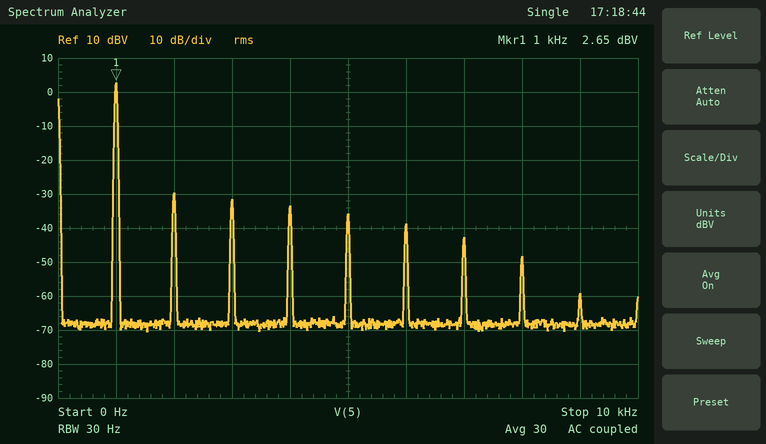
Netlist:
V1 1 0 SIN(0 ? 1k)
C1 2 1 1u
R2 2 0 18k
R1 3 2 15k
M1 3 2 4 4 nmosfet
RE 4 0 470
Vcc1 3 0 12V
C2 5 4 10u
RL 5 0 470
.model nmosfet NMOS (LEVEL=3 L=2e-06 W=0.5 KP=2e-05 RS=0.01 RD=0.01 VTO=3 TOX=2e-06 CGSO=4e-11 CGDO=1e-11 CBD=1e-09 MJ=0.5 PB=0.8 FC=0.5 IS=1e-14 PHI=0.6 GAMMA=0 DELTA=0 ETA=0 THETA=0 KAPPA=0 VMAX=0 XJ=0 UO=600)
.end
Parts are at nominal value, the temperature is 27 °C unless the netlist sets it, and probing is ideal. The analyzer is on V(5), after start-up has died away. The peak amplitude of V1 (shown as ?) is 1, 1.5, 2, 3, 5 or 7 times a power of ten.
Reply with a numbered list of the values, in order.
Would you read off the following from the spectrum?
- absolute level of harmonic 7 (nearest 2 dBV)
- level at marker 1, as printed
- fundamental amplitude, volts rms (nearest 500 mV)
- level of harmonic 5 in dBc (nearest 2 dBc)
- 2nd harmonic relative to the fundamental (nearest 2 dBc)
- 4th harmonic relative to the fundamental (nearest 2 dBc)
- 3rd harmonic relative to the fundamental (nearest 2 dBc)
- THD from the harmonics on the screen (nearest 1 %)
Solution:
1. -42 dBV
2. 2.65 dBV
3. 1.5 V
4. -38 dBc
5. -32 dBc
6. -36 dBc
7. -34 dBc
8. 4 %
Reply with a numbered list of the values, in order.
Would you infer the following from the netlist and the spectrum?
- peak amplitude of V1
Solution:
1. 2 V
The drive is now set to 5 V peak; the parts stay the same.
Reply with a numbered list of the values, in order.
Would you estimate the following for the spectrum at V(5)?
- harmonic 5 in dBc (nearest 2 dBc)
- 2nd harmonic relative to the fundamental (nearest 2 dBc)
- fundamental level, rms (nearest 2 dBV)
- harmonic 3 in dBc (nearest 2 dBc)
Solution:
1. -28 dBc
2. -10 dBc
3. 8 dBV
4. -22 dBc
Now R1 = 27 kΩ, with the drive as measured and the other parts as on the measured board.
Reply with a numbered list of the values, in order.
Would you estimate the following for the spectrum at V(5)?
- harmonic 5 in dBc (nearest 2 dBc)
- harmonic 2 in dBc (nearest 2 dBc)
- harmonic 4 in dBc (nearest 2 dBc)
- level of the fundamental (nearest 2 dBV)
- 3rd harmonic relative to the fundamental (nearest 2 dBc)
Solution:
1. -30 dBc
2. -12 dBc
3. -42 dBc
4. 0 dBV
5. -22 dBc
